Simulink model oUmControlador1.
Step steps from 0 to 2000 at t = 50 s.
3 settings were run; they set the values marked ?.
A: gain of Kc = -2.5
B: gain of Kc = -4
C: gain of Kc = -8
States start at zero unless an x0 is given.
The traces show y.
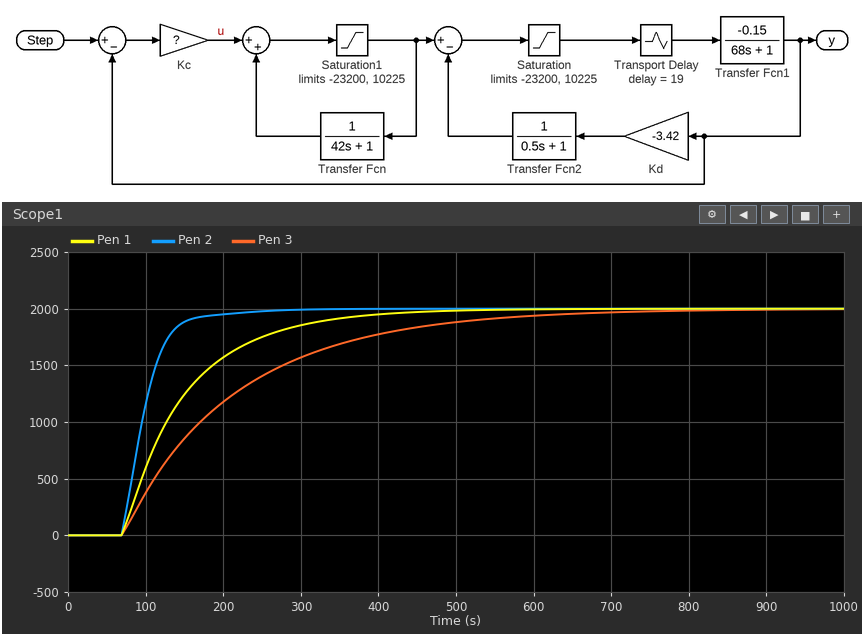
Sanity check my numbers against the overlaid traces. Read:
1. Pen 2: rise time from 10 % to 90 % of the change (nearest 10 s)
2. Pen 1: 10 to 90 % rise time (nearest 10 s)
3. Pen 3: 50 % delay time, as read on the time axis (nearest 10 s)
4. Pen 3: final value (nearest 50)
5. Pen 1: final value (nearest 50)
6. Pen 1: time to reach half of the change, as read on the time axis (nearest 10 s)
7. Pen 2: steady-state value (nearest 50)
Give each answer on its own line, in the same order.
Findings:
60 s
190 s
170 s
2000
2000
130 s
2000
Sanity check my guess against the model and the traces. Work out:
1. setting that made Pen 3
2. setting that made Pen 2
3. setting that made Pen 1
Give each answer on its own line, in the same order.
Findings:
A
C
B
